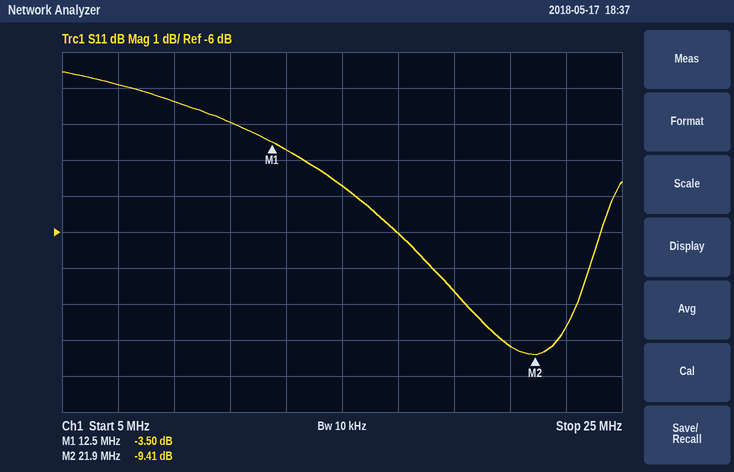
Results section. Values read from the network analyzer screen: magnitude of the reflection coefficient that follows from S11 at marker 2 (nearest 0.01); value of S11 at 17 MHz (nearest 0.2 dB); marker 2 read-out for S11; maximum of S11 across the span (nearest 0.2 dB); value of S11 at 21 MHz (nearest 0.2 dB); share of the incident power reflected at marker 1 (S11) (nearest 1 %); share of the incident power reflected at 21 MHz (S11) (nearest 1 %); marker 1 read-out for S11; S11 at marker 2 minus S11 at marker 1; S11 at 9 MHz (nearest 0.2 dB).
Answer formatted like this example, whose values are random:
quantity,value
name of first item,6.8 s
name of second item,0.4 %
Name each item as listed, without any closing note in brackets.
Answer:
quantity,value
magnitude of the reflection coefficient that follows from S11 at marker 2,0.34
value of S11 at 17 MHz,-6.0 dB
marker 2 read-out for S11,-9.41 dB
maximum of S11 across the span,-1.6 dB
value of S11 at 21 MHz,-9.2 dB
share of the incident power reflected at marker 1 (S11),45 %
share of the incident power reflected at 21 MHz (S11),12 %
marker 1 read-out for S11,-3.50 dB
S11 at marker 2 minus S11 at marker 1,-5.91 dB
S11 at 9 MHz,-2.4 dB
